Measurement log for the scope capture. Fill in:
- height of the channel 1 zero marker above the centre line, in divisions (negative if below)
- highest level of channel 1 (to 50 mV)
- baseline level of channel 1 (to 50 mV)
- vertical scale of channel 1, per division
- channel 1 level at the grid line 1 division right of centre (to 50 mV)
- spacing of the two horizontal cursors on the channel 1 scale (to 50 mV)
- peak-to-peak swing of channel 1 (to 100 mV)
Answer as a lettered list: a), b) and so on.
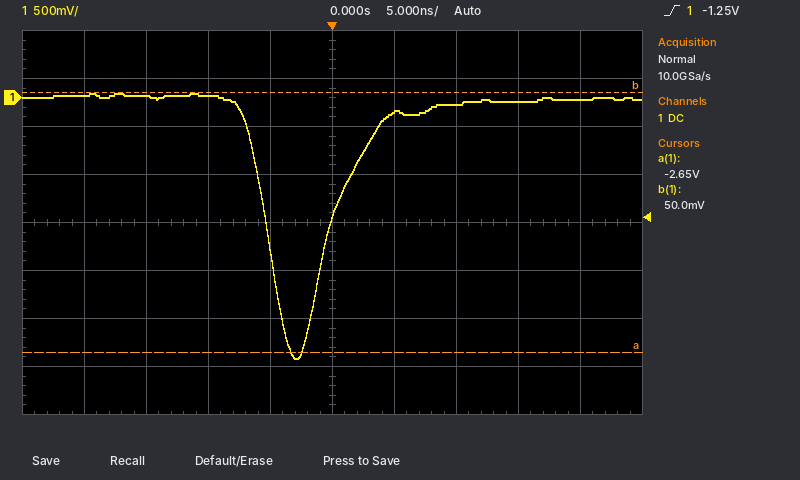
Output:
a) +2.6 div
b) 50 mV
c) 0 mV
d) 500 mV
e) -150 mV
f) 2.70 V
g) 2.80 V
